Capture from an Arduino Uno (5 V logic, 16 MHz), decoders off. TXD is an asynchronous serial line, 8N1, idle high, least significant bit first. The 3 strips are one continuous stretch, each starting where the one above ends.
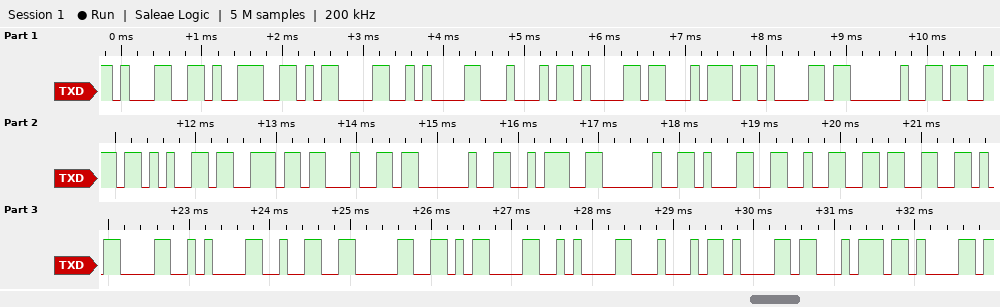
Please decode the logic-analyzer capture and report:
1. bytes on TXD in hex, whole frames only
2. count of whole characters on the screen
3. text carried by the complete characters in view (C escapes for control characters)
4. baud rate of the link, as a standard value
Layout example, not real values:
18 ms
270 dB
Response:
31 39 0D 0A 44 61 74 61 20 73 65 6E 64 20 3A 20 31 32 33 0D 0A 32 30 0D 0A 44 61 74 61
29
"19\r\nData send : 123\r\n20\r\nData"
9600 baud
